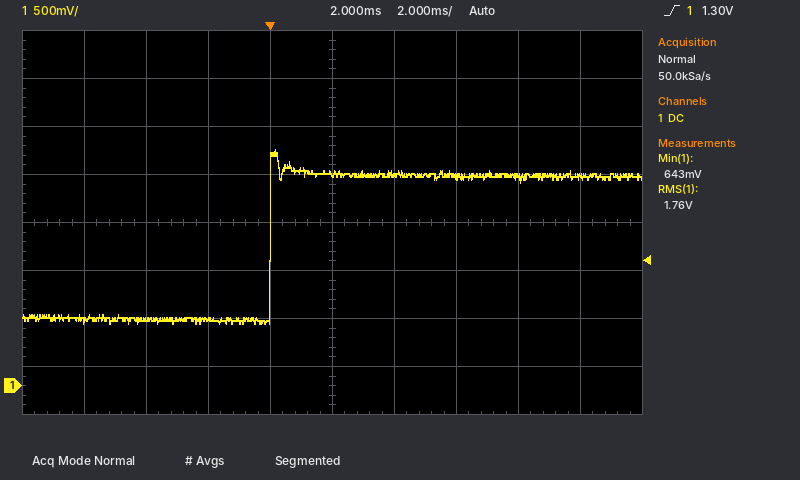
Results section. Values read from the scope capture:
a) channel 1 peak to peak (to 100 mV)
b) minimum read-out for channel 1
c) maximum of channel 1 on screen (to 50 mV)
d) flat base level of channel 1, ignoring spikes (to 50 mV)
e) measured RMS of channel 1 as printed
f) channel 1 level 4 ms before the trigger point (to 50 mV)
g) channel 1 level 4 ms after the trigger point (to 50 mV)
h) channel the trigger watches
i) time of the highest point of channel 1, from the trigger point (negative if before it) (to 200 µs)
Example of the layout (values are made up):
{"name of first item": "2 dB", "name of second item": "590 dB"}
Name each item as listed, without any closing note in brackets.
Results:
{"channel 1 peak to peak": "1.80 V", "minimum read-out for channel 1": "643 mV", "maximum of channel 1 on screen": "2.45 V", "flat base level of channel 1, ignoring spikes": "700 mV", "measured RMS of channel 1 as printed": "1.76 V", "channel 1 level 4 ms before the trigger point": "700 mV", "channel 1 level 4 ms after the trigger point": "2.20 V", "channel the trigger watches": "channel 1", "time of the highest point of channel 1, from the trigger point (negative if before it)": "+200 µs"}
